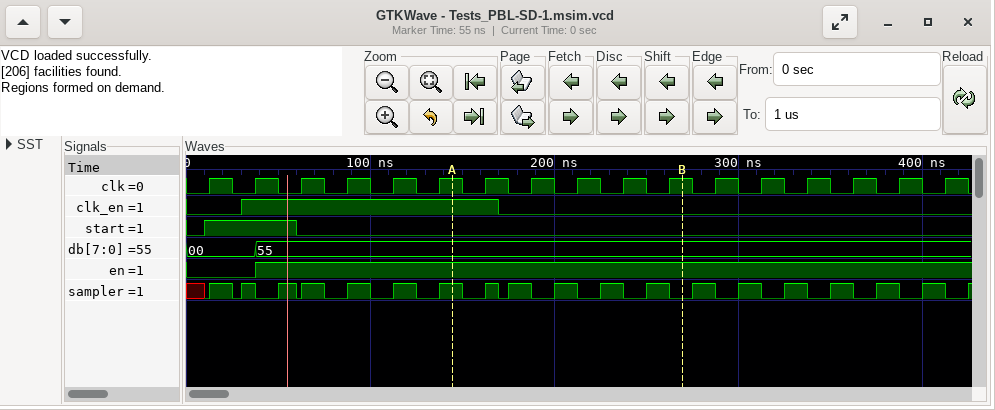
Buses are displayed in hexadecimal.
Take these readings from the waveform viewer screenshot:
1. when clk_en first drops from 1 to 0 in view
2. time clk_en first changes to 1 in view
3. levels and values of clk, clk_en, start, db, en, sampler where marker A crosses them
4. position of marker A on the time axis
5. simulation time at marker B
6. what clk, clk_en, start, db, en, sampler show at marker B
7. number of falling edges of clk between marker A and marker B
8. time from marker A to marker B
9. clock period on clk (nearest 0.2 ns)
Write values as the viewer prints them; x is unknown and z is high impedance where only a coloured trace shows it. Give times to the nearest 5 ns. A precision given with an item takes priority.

170 ns
30 ns
clk=1, clk_en=1, start=0, db=55, en=1, sampler=1
145 ns
270 ns
clk=1, clk_en=0, start=0, db=55, en=1, sampler=0
5
125 ns
25 ns
